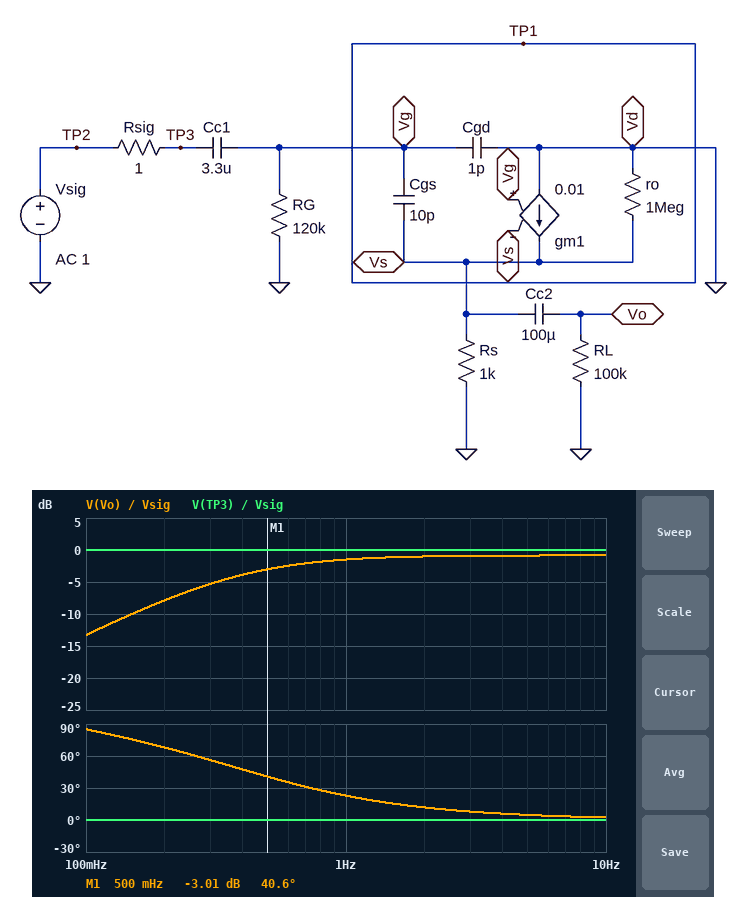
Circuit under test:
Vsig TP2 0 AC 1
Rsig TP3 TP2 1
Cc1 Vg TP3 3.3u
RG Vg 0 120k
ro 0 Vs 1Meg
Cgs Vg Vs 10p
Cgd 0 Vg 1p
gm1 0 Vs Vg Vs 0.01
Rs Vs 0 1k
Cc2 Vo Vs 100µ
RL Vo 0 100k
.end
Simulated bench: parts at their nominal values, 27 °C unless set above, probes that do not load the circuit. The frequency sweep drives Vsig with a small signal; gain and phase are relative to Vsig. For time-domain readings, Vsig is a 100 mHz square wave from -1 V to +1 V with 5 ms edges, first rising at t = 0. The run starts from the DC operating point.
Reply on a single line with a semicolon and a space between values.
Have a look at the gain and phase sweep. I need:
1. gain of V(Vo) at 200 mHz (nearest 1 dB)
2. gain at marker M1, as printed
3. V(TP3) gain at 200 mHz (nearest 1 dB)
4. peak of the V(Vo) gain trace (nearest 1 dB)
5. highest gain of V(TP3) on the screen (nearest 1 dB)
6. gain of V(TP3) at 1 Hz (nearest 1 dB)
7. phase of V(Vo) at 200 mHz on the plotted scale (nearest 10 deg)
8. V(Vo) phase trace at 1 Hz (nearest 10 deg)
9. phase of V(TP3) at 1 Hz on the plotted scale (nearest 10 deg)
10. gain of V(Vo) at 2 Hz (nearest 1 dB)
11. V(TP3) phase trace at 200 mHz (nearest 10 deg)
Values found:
-8 dB; -3.01 dB; 0 dB; -1 dB; 0 dB; 0 dB; 70 deg; 20 deg; 0 deg; -1 dB; 0 deg
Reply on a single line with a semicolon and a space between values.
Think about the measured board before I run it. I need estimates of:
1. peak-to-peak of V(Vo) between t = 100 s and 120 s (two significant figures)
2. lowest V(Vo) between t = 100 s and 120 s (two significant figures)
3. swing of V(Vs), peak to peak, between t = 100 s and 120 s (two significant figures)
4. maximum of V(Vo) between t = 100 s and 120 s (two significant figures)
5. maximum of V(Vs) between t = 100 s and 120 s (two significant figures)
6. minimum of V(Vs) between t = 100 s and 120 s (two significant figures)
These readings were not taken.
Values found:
3.7 V; -1.8 V; 3.6 V; 1.8 V; 1.8 V; -1.8 V
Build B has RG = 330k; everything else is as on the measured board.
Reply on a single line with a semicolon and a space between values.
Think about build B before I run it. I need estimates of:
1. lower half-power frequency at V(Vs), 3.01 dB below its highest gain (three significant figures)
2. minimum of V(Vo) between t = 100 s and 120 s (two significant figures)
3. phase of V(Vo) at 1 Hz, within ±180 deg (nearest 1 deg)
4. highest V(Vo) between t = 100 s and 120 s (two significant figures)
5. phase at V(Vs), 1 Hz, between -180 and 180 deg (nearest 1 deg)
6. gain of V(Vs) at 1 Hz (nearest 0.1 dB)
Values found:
146 mHz; -1.9 V; 9 deg; 1.9 V; 8 deg; -0.9 dB
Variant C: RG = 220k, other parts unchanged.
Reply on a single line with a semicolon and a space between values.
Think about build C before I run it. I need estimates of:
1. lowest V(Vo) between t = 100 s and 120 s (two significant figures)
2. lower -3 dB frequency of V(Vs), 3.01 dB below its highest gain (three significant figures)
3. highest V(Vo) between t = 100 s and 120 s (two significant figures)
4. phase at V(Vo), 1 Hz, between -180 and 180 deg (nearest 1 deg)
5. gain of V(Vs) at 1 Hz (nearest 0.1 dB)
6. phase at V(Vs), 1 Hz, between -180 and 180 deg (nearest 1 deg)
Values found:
-1.9 V; 219 mHz; 1.9 V; 13 deg; -1.0 dB; 12 deg
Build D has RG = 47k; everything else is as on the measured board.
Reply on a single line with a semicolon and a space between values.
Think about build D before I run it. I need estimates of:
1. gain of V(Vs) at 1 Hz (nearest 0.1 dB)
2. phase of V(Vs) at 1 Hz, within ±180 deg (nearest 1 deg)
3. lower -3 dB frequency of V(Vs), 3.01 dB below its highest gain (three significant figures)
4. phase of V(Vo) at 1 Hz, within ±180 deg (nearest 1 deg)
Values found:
-4.0 dB; 46 deg; 1.03 Hz; 47 deg
